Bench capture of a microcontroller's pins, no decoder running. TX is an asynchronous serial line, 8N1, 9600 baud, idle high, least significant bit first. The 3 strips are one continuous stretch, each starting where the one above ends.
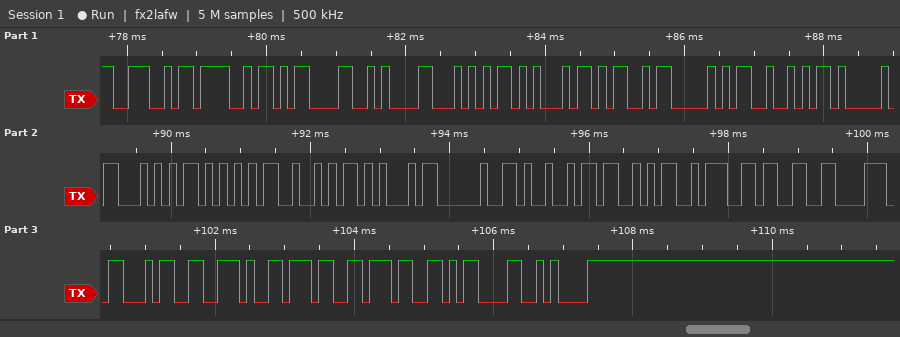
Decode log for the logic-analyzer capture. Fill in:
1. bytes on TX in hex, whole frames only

4E 4F 0D 0A 54 45 4D 50 52 41 54 55 52 45 20 49 53 3A 33 38 34 2E 37 37 0D 0A
